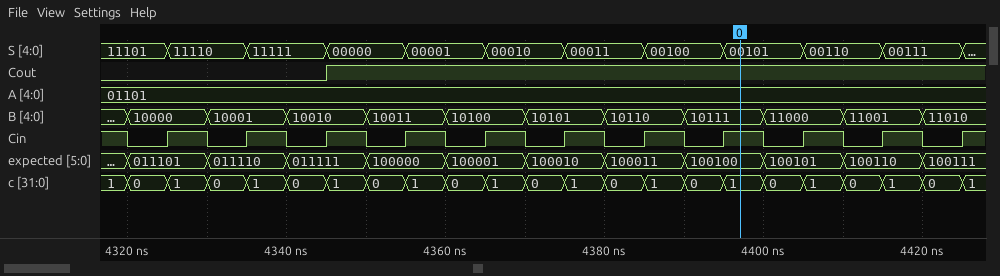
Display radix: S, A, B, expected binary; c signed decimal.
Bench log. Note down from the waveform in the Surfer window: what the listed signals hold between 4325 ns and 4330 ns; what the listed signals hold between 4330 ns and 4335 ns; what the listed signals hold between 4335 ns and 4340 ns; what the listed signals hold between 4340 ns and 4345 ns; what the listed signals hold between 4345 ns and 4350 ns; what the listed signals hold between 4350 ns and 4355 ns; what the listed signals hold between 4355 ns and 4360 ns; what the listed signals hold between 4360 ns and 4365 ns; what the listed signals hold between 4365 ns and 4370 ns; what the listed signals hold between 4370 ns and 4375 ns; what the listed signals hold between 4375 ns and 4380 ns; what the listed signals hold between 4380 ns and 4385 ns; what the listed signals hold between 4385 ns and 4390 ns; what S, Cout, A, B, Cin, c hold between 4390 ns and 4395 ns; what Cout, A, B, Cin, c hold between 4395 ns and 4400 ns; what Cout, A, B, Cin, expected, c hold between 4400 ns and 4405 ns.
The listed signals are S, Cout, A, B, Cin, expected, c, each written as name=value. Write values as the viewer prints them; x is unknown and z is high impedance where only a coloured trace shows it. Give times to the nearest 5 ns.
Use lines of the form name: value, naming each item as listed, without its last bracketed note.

what the listed signals hold between 4325 ns and 4330 ns: S=11110, Cout=0, A=01101, B=10000, Cin=1, expected=011101, c=1
what the listed signals hold between 4330 ns and 4335 ns: S=11110, Cout=0, A=01101, B=10001, Cin=0, expected=011110, c=0
what the listed signals hold between 4335 ns and 4340 ns: S=11111, Cout=0, A=01101, B=10001, Cin=1, expected=011110, c=1
what the listed signals hold between 4340 ns and 4345 ns: S=11111, Cout=0, A=01101, B=10010, Cin=0, expected=011111, c=0
what the listed signals hold between 4345 ns and 4350 ns: S=00000, Cout=1, A=01101, B=10010, Cin=1, expected=011111, c=1
what the listed signals hold between 4350 ns and 4355 ns: S=00000, Cout=1, A=01101, B=10011, Cin=0, expected=100000, c=0
what the listed signals hold between 4355 ns and 4360 ns: S=00001, Cout=1, A=01101, B=10011, Cin=1, expected=100000, c=1
what the listed signals hold between 4360 ns and 4365 ns: S=00001, Cout=1, A=01101, B=10100, Cin=0, expected=100001, c=0
what the listed signals hold between 4365 ns and 4370 ns: S=00010, Cout=1, A=01101, B=10100, Cin=1, expected=100001, c=1
what the listed signals hold between 4370 ns and 4375 ns: S=00010, Cout=1, A=01101, B=10101, Cin=0, expected=100010, c=0
what the listed signals hold between 4375 ns and 4380 ns: S=00011, Cout=1, A=01101, B=10101, Cin=1, expected=100010, c=1
what the listed signals hold between 4380 ns and 4385 ns: S=00011, Cout=1, A=01101, B=10110, Cin=0, expected=100011, c=0
what the listed signals hold between 4385 ns and 4390 ns: S=00100, Cout=1, A=01101, B=10110, Cin=1, expected=100011, c=1
what S, Cout, A, B, Cin, c hold between 4390 ns and 4395 ns: S=00100, Cout=1, A=01101, B=10111, Cin=0, c=0
what Cout, A, B, Cin, c hold between 4395 ns and 4400 ns: Cout=1, A=01101, B=10111, Cin=1, c=1
what Cout, A, B, Cin, expected, c hold between 4400 ns and 4405 ns: Cout=1, A=01101, B=11000, Cin=0, expected=100101, c=0
